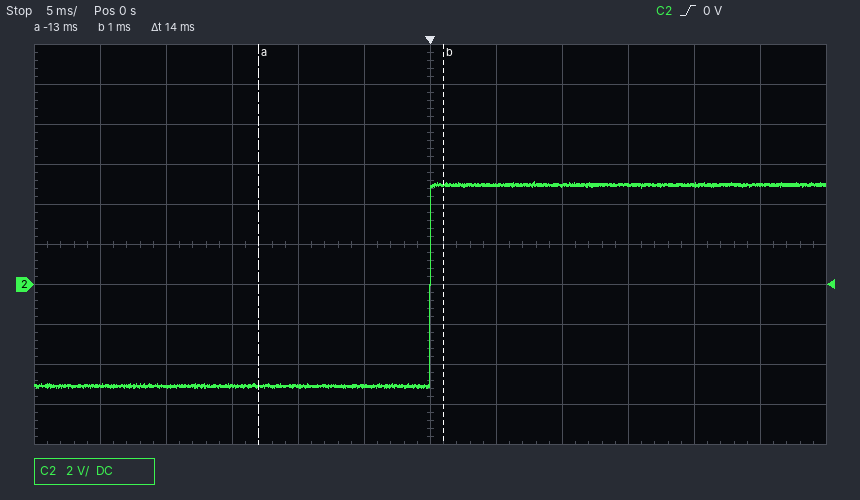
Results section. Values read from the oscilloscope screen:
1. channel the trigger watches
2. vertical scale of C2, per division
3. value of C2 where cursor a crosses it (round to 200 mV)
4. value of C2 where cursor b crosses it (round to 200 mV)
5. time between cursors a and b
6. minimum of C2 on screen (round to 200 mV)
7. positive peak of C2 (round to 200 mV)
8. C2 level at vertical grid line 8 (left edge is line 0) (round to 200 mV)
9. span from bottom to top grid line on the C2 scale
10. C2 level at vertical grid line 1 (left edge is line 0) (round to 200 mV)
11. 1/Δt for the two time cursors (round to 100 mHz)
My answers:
C2
2 V
-5.0 V
5.0 V
14 ms
-5.2 V
5.2 V
5.0 V
20 V
-5.0 V
71.4 Hz
